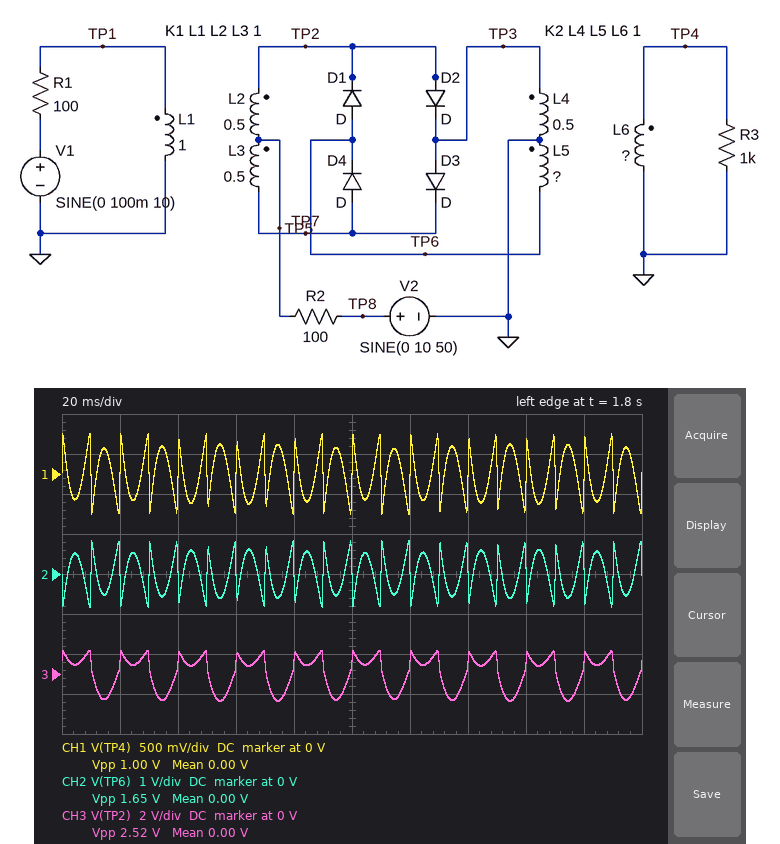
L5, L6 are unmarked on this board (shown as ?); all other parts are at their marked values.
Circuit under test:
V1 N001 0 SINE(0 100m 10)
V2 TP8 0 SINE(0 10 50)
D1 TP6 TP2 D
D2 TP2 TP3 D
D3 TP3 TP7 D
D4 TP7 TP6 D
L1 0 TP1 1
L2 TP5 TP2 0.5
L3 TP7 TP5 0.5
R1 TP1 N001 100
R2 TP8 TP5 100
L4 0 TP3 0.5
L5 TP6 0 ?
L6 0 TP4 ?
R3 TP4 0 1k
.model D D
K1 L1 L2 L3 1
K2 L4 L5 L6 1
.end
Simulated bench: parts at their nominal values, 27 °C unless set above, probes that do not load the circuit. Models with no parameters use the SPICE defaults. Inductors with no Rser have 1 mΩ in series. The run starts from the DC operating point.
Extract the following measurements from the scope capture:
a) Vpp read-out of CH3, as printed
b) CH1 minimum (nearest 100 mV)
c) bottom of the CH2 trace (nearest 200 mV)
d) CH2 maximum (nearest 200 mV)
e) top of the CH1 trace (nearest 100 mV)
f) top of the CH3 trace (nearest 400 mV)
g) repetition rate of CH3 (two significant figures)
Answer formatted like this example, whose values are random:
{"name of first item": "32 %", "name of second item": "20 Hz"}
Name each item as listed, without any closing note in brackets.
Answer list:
{"Vpp read-out of CH3, as printed": "2.52 V", "CH1 minimum": "-500 mV", "bottom of the CH2 trace": "-800 mV", "CH2 maximum": "800 mV", "top of the CH1 trace": "500 mV", "top of the CH3 trace": "1.2 V", "repetition rate of CH3": "50 Hz"}
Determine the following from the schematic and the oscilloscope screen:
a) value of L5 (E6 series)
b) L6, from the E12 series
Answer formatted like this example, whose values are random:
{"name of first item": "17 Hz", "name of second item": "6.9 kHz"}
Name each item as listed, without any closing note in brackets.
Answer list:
{"value of L5": "1.5 H", "L6, from the E12 series": "560 mH"}
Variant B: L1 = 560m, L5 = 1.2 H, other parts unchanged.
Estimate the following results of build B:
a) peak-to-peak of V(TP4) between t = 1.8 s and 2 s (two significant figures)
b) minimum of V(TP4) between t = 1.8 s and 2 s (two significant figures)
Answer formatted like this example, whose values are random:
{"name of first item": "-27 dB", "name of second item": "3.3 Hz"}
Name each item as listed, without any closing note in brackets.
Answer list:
{"peak-to-peak of V(TP4) between t = 1.8 s and 2 s": "1.1 V", "minimum of V(TP4) between t = 1.8 s and 2 s": "-560 mV"}
